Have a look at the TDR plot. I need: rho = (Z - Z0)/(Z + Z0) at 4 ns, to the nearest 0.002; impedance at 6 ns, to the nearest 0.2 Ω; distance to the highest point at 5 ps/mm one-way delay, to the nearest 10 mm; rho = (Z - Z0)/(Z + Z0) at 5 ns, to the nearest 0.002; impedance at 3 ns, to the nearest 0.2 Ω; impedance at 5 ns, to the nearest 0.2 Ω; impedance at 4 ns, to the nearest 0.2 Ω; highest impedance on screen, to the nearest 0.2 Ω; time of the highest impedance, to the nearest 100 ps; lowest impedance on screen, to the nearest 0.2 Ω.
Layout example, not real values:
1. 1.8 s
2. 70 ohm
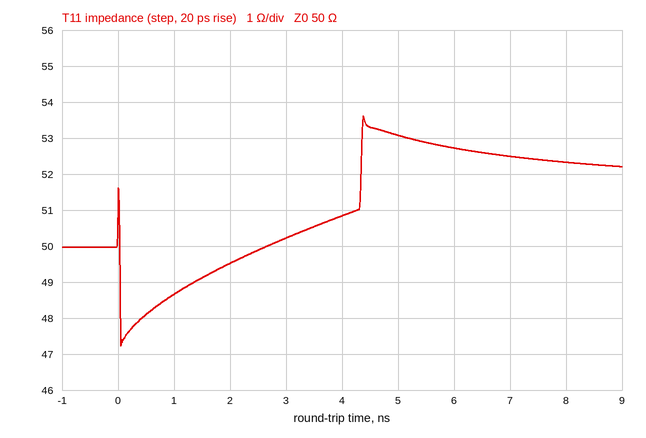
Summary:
1. +0.008
2. 52.8 Ω
3. 440 mm
4. +0.030
5. 50.2 Ω
6. 53.0 Ω
7. 50.8 Ω
8. 53.6 Ω
9. 4.4 ns
10. 47.2 Ω
